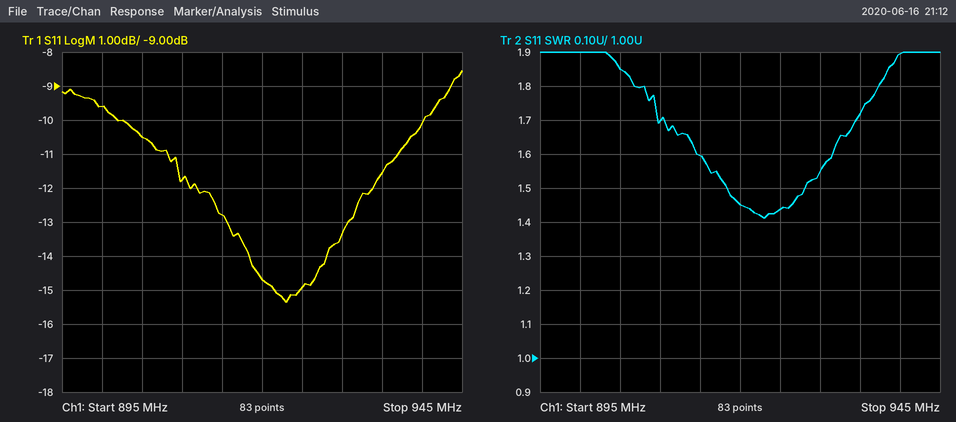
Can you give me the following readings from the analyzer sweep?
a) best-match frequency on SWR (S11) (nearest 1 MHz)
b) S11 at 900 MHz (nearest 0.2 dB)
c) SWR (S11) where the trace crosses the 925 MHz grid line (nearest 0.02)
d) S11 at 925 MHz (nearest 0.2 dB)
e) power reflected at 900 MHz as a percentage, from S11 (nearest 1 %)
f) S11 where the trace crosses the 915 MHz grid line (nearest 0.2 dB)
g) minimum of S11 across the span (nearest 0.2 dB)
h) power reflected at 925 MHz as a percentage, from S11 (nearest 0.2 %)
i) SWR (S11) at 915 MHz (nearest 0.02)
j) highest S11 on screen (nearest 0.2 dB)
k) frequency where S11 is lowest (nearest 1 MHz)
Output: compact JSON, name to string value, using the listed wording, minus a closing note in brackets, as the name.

{"best-match frequency on SWR (S11)": "923 MHz", "S11 at 900 MHz": "-9.6 dB", "SWR (S11) where the trace crosses the 925 MHz grid line": "1.44", "S11 at 925 MHz": "-15.0 dB", "power reflected at 900 MHz as a percentage, from S11": "11 %", "S11 where the trace crosses the 915 MHz grid line": "-12.8 dB", "minimum of S11 across the span": "-15.4 dB", "power reflected at 925 MHz as a percentage, from S11": "3.2 %", "SWR (S11) at 915 MHz": "1.60", "highest S11 on screen": "-8.6 dB", "frequency where S11 is lowest": "923 MHz"}
